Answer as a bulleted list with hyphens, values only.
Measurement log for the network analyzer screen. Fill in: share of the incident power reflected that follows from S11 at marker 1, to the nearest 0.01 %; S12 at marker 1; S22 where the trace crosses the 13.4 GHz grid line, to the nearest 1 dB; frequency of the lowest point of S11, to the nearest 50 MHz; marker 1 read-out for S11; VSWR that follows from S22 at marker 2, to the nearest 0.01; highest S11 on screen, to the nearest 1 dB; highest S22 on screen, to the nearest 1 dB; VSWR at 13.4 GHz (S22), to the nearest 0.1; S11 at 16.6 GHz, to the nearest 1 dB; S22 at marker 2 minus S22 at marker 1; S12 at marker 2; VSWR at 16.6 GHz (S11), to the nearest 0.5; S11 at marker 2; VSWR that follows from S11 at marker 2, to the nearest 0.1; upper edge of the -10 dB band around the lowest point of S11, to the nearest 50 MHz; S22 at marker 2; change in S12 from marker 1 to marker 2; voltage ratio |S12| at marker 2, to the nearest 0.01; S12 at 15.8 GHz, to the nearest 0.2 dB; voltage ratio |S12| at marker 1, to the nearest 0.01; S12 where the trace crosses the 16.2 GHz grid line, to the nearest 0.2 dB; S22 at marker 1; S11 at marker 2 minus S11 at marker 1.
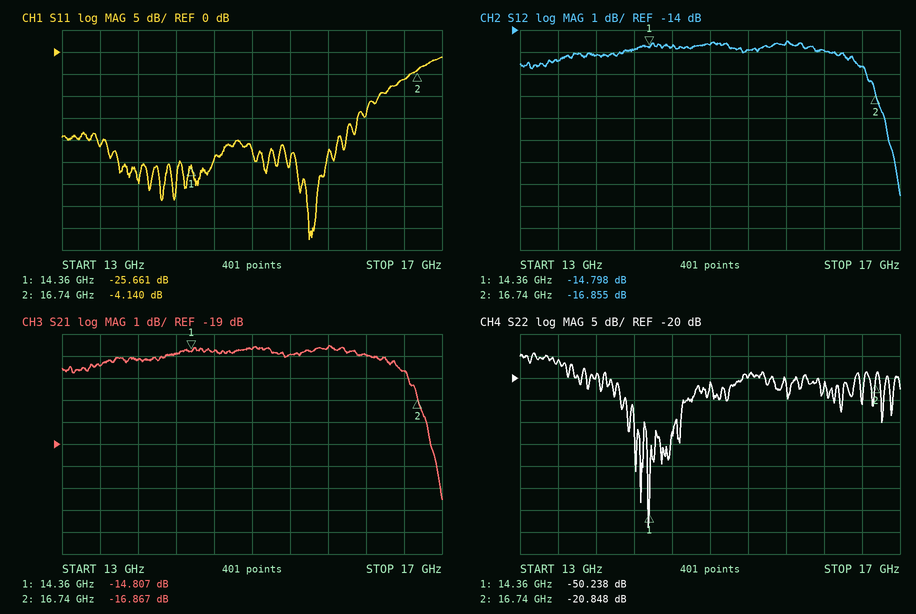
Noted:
- 0.27 %
- -14.798 dB
- -16 dB
- 15.60 GHz
- -25.661 dB
- 1.20
- -1 dB
- -14 dB
- 1.4
- -6 dB
- 29.390 dB
- -16.855 dB
- 3.0
- -4.140 dB
- 4.3
- 16.35 GHz
- -20.848 dB
- -2.057 dB
- 0.14
- -14.6 dB
- 0.18
- -15.0 dB
- -50.238 dB
- 21.521 dB
